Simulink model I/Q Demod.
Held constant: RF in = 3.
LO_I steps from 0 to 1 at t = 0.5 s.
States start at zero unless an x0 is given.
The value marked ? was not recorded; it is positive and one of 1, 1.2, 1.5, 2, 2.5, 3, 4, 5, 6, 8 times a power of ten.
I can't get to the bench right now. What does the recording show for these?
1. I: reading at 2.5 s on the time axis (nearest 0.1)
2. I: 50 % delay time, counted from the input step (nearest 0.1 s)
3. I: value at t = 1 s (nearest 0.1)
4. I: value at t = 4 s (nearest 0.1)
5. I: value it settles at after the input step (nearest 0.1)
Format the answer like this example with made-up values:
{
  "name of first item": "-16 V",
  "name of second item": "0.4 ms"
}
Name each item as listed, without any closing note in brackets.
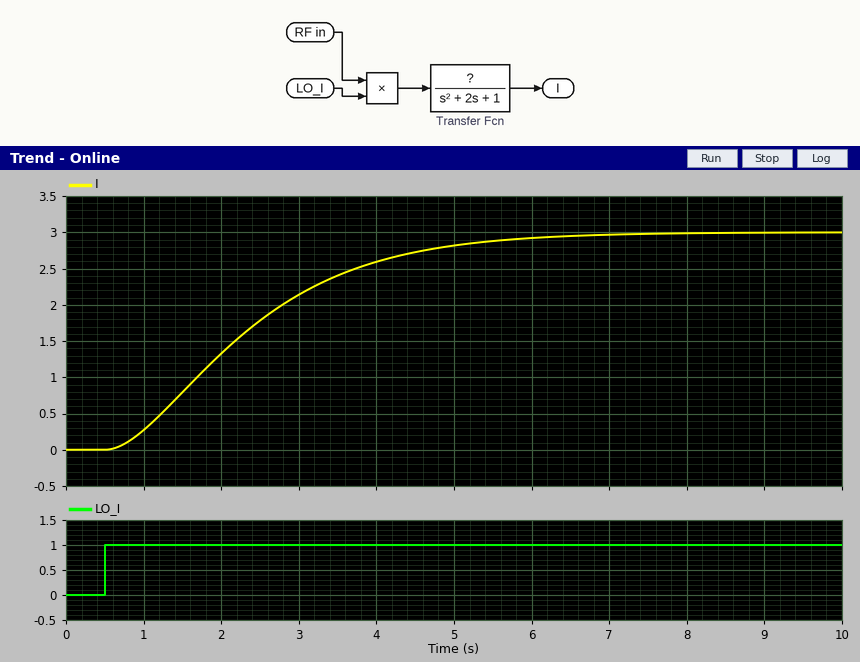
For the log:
{
  "I: reading at 2.5 s on the time axis": "1.8",
  "I: 50 % delay time, counted from the input step": "1.7 s",
  "I: value at t = 1 s": "0.3",
  "I: value at t = 4 s": "2.6",
  "I: value it settles at after the input step": "3.0"
}
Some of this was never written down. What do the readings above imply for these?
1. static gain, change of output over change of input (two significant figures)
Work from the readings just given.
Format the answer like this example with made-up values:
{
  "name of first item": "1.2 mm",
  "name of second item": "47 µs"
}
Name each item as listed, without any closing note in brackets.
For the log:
{
  "static gain, change of output over change of input": "3.0"
}
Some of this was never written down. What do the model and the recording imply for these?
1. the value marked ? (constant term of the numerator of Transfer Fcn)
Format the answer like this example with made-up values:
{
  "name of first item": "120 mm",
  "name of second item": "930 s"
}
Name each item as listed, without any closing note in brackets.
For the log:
{
  "the value marked ?": "1"
}
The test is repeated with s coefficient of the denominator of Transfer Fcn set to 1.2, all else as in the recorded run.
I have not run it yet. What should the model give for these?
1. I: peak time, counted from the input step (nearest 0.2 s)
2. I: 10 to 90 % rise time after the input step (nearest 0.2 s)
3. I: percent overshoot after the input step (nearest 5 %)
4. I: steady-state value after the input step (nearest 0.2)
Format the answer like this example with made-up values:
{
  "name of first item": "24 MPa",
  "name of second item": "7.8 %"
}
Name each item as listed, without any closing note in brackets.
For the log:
{
  "I: peak time, counted from the input step": "4.0 s",
  "I: 10 to 90 % rise time after the input step": "1.8 s",
  "I: percent overshoot after the input step": "10 %",
  "I: steady-state value after the input step": "3.0"
}
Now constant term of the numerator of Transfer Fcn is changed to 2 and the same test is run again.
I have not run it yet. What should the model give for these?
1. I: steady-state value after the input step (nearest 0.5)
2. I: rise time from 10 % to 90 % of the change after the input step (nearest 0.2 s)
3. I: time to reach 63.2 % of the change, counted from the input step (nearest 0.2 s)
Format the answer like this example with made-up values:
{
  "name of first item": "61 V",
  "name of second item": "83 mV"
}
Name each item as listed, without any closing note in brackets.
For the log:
{
  "I: steady-state value after the input step": "6.0",
  "I: rise time from 10 % to 90 % of the change after the input step": "3.4 s",
  "I: time to reach 63.2 % of the change, counted from the input step": "2.2 s"
}
